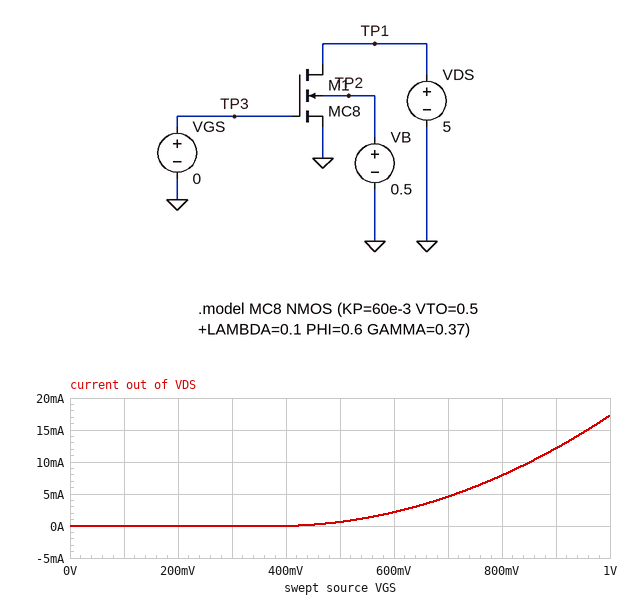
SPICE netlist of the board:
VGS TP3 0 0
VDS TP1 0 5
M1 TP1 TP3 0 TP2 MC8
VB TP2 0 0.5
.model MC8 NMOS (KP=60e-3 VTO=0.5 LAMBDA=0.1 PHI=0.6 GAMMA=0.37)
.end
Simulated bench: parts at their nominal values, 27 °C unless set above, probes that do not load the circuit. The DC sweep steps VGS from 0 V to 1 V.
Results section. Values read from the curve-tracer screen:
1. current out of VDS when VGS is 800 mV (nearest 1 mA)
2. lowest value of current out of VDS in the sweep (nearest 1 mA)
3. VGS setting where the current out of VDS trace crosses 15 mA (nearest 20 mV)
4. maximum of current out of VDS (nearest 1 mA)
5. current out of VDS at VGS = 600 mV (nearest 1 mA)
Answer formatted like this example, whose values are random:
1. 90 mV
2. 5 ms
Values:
1. 8 mA
2. 0 A
3. 960 mV
4. 17 mA
5. 2 mA
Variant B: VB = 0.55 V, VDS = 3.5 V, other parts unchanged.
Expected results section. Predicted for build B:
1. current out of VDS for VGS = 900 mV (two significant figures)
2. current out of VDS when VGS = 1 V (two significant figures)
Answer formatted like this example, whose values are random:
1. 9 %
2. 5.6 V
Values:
1. 11 mA
2. 16 mA
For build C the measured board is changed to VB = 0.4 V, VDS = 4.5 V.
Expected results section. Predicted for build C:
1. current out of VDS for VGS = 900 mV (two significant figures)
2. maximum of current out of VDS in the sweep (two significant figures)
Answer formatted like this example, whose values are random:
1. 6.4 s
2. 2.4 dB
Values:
1. 11 mA
2. 15 mA
